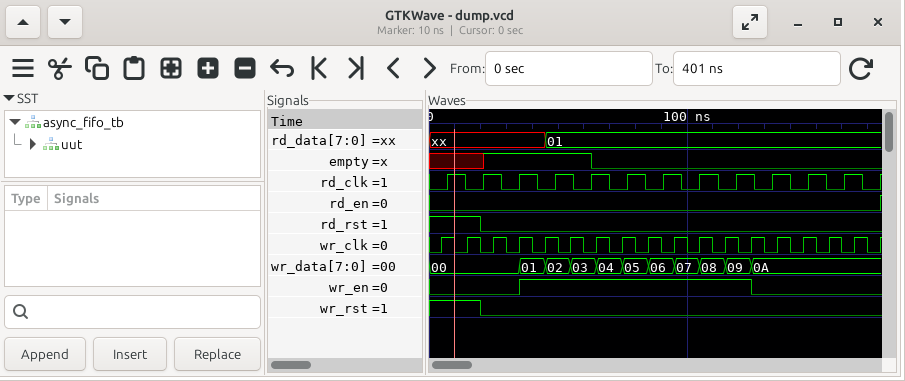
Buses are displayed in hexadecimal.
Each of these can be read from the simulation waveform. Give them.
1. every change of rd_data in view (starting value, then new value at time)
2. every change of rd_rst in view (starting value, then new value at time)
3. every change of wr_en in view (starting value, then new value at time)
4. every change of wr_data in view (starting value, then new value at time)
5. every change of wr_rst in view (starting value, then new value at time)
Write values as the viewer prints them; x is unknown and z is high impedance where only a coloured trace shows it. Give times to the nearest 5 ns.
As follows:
xx, 01 at 45 ns
1, 0 at 20 ns
0, 1 at 35 ns, 0 at 125 ns
00, 01 at 35 ns, 02 at 45 ns, 03 at 55 ns, 04 at 65 ns, 05 at 75 ns, 06 at 85 ns, 07 at 95 ns, 08 at 105 ns, 09 at 115 ns, 0A at 125 ns
1, 0 at 20 ns
